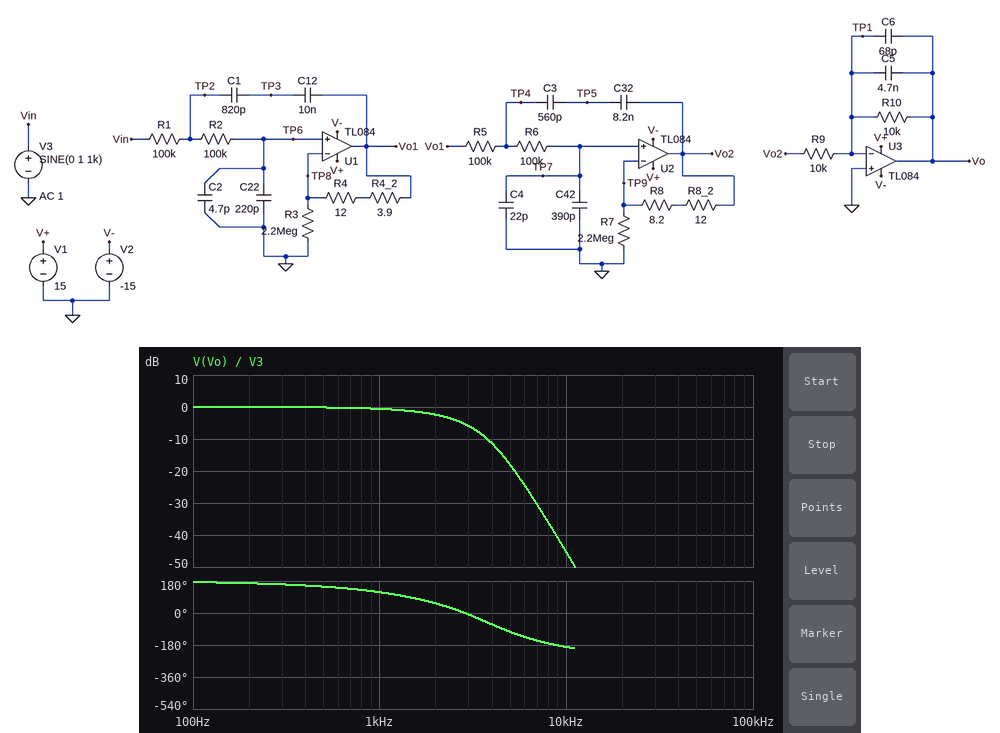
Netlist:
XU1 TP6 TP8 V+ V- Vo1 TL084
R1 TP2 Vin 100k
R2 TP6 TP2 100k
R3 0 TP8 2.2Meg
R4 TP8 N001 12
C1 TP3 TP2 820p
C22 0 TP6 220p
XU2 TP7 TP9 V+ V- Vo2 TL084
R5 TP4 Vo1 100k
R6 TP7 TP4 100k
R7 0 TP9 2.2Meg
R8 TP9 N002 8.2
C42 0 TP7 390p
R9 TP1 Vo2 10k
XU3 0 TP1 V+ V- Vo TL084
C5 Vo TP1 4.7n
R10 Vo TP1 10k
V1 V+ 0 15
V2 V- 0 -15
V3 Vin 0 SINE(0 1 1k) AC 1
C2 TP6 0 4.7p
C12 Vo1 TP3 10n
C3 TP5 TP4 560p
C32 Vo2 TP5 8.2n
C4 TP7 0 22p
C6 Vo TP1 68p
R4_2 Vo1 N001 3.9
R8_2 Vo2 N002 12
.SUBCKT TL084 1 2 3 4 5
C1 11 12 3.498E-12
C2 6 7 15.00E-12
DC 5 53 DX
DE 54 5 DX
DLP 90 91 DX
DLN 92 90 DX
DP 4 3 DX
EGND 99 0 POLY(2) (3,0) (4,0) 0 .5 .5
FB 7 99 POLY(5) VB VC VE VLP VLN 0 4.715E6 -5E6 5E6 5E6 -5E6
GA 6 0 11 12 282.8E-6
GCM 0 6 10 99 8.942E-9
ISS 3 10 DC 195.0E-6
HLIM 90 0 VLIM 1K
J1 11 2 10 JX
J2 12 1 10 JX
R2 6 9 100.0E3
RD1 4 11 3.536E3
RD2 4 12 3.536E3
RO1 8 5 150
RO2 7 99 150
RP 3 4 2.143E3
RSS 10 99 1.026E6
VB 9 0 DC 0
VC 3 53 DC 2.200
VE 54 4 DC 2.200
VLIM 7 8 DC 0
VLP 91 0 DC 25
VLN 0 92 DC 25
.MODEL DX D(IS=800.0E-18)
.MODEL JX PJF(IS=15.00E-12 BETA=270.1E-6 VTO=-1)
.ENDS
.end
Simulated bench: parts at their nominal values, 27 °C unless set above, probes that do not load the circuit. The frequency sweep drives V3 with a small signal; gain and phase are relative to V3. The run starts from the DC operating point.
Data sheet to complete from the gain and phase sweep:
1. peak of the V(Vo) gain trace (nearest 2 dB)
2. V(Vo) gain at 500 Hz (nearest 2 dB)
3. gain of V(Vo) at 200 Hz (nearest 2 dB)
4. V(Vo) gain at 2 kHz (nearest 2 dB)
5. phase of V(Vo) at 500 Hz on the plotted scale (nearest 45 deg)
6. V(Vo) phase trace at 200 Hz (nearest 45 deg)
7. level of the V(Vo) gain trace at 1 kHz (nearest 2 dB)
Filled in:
0 dB
0 dB
0 dB
-2 dB
135 deg
180 deg
0 dB
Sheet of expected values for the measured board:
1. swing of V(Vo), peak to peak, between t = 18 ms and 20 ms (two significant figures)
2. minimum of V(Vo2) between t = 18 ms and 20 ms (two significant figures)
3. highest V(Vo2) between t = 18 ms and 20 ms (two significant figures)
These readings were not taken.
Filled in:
1.9 V
-980 mV
980 mV
